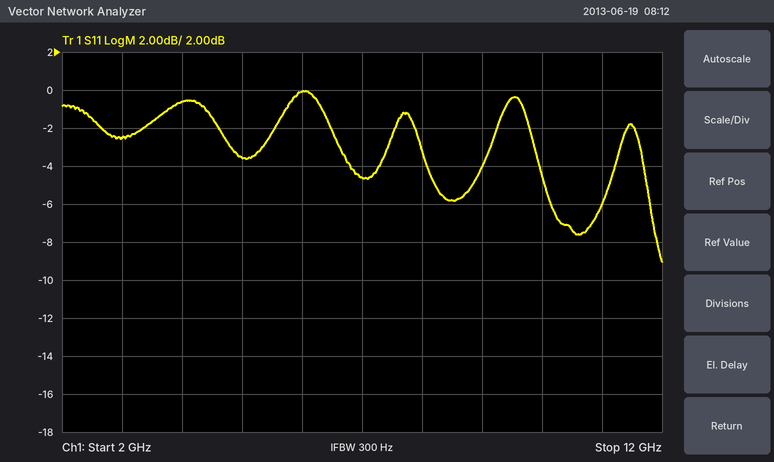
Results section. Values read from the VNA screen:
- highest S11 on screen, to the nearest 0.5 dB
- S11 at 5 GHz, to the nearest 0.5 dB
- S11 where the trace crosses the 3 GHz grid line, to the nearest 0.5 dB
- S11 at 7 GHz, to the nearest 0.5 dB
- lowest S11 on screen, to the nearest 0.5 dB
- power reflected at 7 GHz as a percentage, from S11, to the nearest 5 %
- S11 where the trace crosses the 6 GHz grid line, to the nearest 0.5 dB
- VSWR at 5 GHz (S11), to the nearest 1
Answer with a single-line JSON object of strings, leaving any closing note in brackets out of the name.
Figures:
{"highest S11 on screen, to the nearest 0.5 dB": "0.0 dB", "S11 at 5 GHz, to the nearest 0.5 dB": "-3.5 dB", "S11 where the trace crosses the 3 GHz grid line, to the nearest 0.5 dB": "-2.5 dB", "S11 at 7 GHz, to the nearest 0.5 dB": "-4.5 dB", "lowest S11 on screen, to the nearest 0.5 dB": "-9.0 dB", "power reflected at 7 GHz as a percentage, from S11, to the nearest 5 %": "35 %", "S11 where the trace crosses the 6 GHz grid line, to the nearest 0.5 dB": "0.0 dB", "VSWR at 5 GHz (S11), to the nearest 1": "5"}
